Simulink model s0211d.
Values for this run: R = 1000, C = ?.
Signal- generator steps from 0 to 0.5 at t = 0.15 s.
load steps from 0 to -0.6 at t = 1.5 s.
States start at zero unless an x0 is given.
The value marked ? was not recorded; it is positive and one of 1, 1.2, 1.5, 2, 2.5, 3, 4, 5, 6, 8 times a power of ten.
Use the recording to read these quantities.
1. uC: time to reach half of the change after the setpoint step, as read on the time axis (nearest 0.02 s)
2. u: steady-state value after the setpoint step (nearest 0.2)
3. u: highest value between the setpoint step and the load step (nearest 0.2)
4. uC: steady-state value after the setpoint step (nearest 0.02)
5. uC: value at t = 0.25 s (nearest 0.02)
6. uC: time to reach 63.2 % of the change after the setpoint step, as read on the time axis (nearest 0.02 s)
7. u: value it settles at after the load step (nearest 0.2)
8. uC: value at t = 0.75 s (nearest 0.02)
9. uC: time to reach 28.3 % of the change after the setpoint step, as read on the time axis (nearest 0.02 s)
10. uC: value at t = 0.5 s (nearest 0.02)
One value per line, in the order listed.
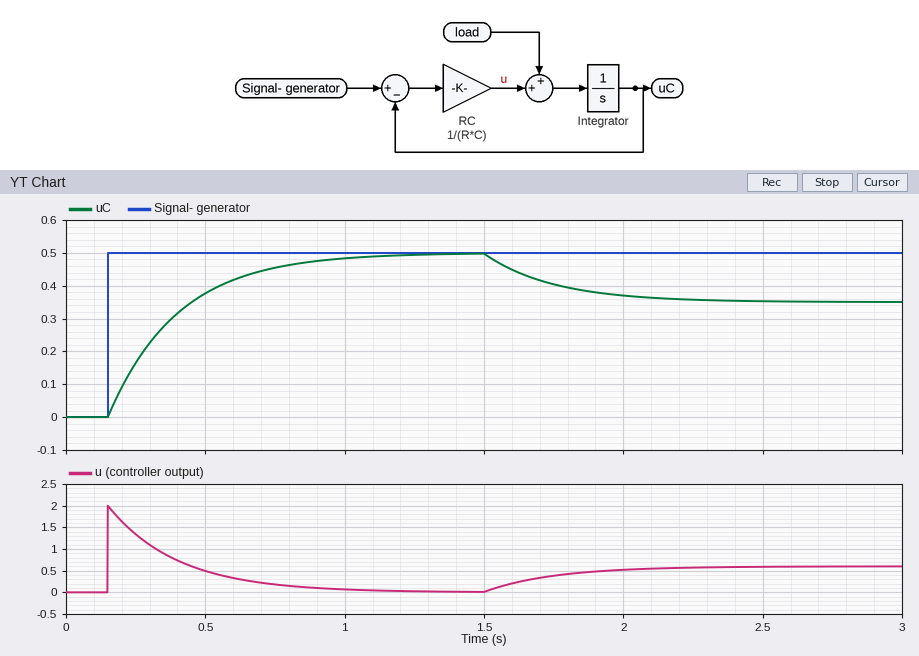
0.32 s
0.0
2.0
0.50
0.16
0.40 s
0.6
0.46
0.24 s
0.38
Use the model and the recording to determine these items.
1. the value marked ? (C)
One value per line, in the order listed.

0.00025
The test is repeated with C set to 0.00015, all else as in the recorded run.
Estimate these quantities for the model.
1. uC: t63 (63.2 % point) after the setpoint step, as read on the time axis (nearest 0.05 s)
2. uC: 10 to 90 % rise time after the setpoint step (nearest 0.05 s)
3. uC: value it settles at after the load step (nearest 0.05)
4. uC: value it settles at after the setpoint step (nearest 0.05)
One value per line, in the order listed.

0.30 s
0.35 s
0.40
0.50
